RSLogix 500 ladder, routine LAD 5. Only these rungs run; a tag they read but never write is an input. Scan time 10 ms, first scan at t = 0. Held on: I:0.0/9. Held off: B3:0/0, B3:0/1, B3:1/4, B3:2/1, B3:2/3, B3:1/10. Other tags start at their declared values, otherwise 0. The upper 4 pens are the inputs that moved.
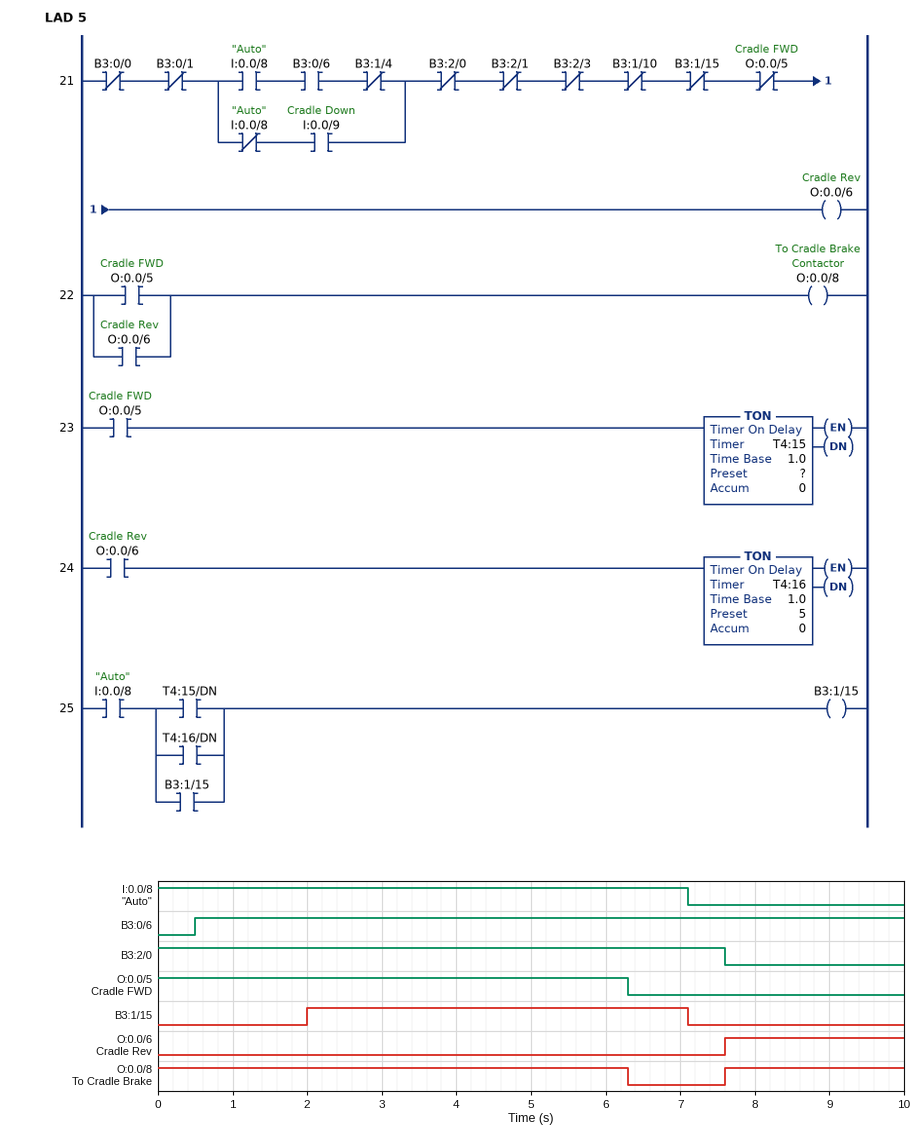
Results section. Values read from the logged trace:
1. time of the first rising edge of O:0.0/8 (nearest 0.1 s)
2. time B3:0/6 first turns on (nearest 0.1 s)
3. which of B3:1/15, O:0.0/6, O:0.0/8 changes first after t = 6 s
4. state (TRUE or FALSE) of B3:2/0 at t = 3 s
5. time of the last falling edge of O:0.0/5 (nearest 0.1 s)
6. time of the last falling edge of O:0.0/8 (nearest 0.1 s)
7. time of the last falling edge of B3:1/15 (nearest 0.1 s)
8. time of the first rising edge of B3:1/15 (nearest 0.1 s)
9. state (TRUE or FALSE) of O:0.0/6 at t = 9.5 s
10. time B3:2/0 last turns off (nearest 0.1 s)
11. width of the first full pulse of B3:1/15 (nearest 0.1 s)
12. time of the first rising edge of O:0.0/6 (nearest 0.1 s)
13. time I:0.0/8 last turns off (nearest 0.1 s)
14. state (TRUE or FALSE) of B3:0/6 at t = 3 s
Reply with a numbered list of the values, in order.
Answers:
1. 7.6 s
2. 0.5 s
3. O:0.0/8
4. TRUE
5. 6.3 s
6. 6.3 s
7. 7.1 s
8. 2.0 s
9. TRUE
10. 7.6 s
11. 5.1 s
12. 7.6 s
13. 7.1 s
14. TRUE
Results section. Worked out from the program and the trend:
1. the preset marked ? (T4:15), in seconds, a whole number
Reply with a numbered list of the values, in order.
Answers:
1. 2 s
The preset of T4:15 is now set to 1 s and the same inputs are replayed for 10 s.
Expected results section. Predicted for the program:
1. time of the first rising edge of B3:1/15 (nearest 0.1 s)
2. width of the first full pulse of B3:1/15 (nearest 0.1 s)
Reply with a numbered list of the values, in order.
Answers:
1. 1.0 s
2. 6.1 s
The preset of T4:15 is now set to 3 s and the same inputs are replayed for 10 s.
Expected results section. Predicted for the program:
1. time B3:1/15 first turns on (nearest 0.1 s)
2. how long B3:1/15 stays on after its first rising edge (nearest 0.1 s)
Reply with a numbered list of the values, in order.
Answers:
1. 3.0 s
2. 4.1 s
